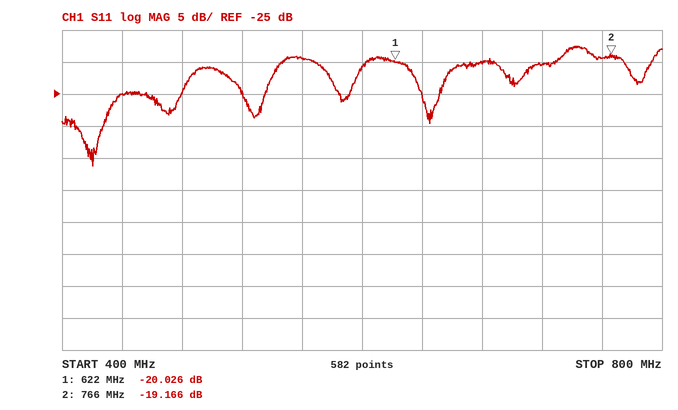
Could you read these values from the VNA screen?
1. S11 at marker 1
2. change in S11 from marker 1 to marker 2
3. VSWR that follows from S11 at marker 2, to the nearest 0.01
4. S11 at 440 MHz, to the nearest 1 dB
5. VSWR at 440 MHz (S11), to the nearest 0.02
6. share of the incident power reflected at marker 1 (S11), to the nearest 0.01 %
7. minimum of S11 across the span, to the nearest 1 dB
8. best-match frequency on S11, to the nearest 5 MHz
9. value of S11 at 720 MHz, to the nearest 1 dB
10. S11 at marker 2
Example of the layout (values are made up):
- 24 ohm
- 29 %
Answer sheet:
- -20.026 dB
- 0.860 dB
- 1.25
- -25 dB
- 1.12
- 0.99 %
- -36 dB
- 420 MHz
- -20 dB
- -19.166 dB
